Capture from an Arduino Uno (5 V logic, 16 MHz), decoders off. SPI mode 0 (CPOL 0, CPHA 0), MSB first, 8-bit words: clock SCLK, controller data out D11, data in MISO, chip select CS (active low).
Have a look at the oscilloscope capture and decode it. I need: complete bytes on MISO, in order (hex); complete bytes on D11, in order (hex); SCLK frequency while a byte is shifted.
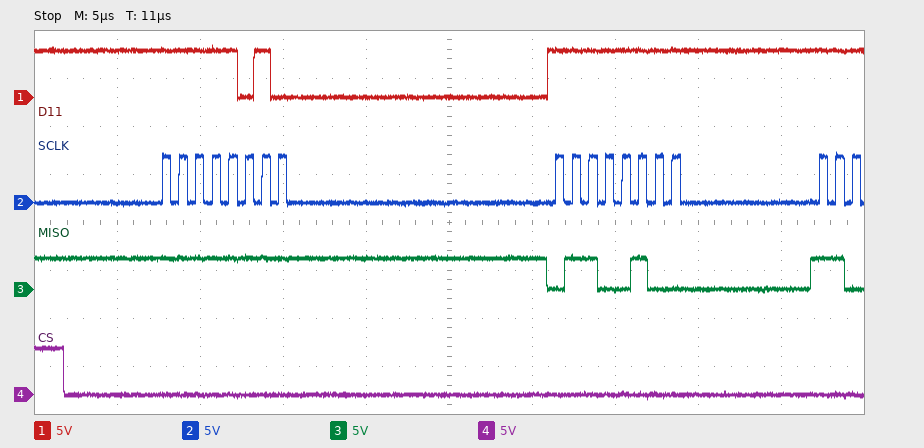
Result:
FF 64
FA FF
1 MHz
